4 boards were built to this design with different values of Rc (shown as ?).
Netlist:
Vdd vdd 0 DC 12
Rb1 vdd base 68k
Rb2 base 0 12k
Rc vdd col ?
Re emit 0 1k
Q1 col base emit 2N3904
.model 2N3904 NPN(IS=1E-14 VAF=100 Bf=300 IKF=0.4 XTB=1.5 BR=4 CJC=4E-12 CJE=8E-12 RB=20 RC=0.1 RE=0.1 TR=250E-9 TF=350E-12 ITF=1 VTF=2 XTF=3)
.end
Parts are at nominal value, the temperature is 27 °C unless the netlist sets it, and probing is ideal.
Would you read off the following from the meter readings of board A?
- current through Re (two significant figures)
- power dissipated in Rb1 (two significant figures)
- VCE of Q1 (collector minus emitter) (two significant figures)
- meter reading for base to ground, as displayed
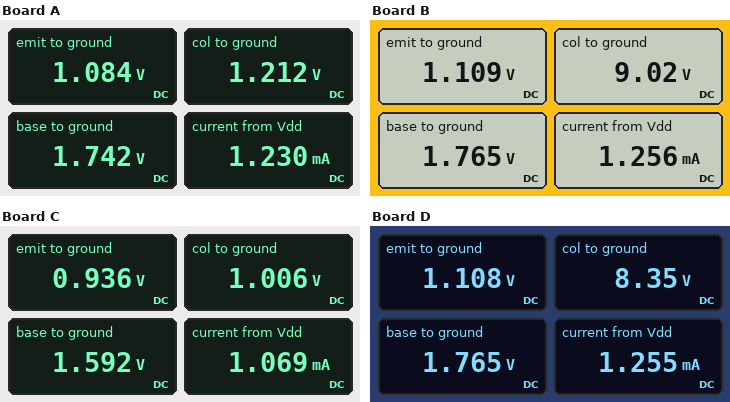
1.1 mA
1.5 mW
130 mV
1.742 V
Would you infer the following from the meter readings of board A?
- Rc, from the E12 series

10 kΩ
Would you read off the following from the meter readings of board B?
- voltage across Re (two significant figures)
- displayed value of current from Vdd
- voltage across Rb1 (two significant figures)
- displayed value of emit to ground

1.1 V
1.256 mA
10 V
1.109 V
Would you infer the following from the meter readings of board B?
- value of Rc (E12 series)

2.7 kΩ
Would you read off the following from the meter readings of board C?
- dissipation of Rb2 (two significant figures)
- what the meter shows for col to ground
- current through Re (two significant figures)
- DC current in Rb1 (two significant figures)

210 µW
1.006 V
940 µA
150 µA
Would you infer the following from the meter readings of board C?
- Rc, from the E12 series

12 kΩ
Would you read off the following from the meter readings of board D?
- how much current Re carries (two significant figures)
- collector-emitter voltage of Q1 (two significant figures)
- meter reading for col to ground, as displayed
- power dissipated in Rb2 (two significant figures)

1.1 mA
7.2 V
8.35 V
260 µW
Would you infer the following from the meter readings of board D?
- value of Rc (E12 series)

3.3 kΩ
